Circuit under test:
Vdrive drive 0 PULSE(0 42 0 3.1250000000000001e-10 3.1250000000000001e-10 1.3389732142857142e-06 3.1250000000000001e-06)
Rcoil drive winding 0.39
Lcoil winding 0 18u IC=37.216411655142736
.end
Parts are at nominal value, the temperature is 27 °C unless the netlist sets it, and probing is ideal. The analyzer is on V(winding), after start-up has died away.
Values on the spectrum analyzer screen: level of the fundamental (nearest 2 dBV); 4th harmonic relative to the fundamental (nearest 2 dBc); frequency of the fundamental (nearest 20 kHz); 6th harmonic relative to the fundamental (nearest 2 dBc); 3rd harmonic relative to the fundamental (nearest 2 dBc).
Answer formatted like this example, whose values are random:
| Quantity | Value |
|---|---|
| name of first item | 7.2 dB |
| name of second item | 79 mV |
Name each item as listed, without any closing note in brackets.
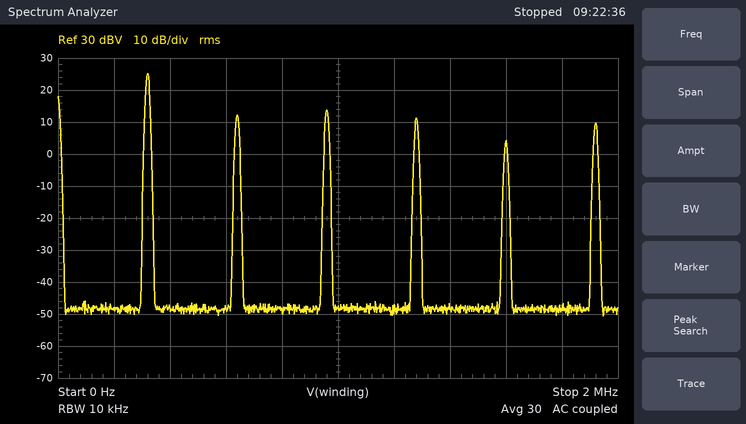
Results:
| Quantity | Value |
|---|---|
| level of the fundamental | 26 dBV |
| 4th harmonic relative to the fundamental | -14 dBc |
| frequency of the fundamental | 320 kHz |
| 6th harmonic relative to the fundamental | -16 dBc |
| 3rd harmonic relative to the fundamental | -12 dBc |
